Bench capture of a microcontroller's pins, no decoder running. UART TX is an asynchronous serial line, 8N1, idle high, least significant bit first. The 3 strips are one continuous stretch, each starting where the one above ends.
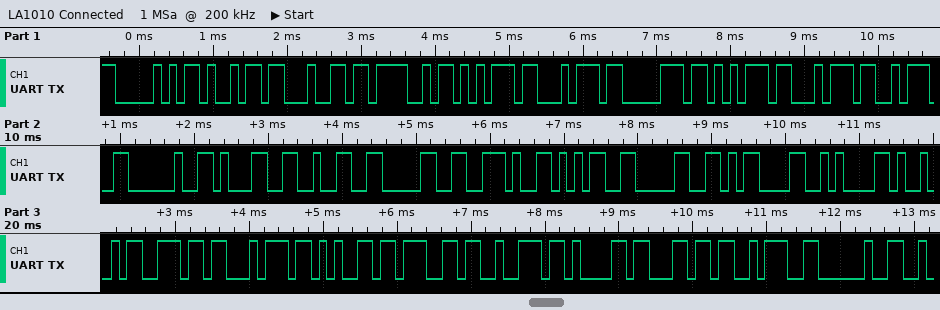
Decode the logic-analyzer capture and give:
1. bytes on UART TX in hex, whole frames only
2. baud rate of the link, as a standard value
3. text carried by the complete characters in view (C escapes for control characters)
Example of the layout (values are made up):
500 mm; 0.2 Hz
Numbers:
50 69 64 4F 75 74 70 75 74 3A 20 31 32 30 2E 35 30 0D 0A 49 6E 74 65 67 72 61 6C 3A 20; 9600 baud; "PidOutput: 120.50\r\nIntegral: "
